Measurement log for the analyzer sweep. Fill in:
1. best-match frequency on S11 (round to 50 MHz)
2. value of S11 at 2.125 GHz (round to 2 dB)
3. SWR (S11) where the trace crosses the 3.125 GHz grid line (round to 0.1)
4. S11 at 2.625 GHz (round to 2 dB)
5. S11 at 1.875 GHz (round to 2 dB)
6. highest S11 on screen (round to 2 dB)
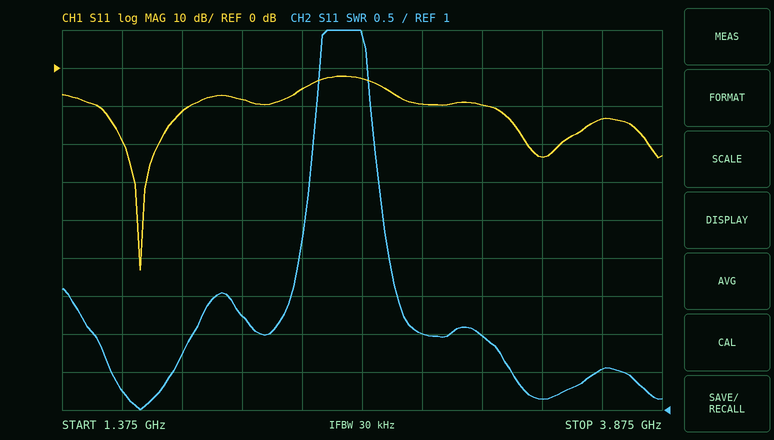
1.70 GHz
-8 dB
2.0
-2 dB
-12 dB
-2 dB
